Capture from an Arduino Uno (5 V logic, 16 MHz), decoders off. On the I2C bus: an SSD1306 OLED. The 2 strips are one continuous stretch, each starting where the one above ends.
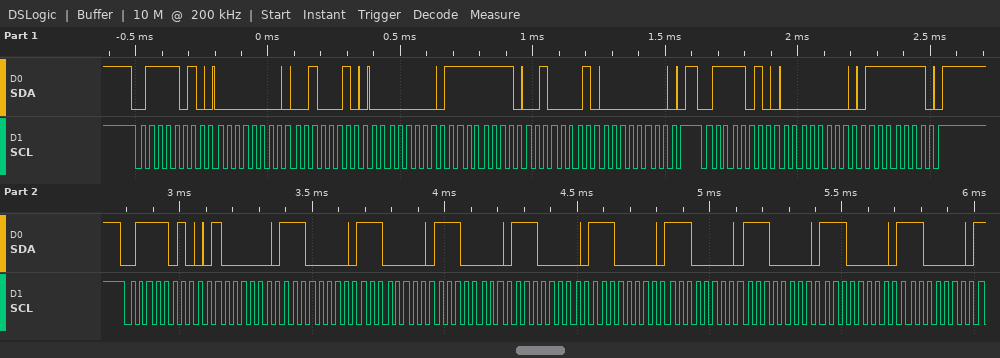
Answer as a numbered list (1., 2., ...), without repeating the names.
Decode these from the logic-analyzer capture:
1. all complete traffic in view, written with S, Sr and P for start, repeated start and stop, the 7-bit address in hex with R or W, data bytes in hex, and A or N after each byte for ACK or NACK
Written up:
1. S 3DW A 00 A 22 A 00 A FF A 21 A 00 A P S 3DW A 00 A 7F A P S 3DW A 40 A E0 A E0 A E0 A E0 A E0 A E0 A E0 A E0 A E0 A
